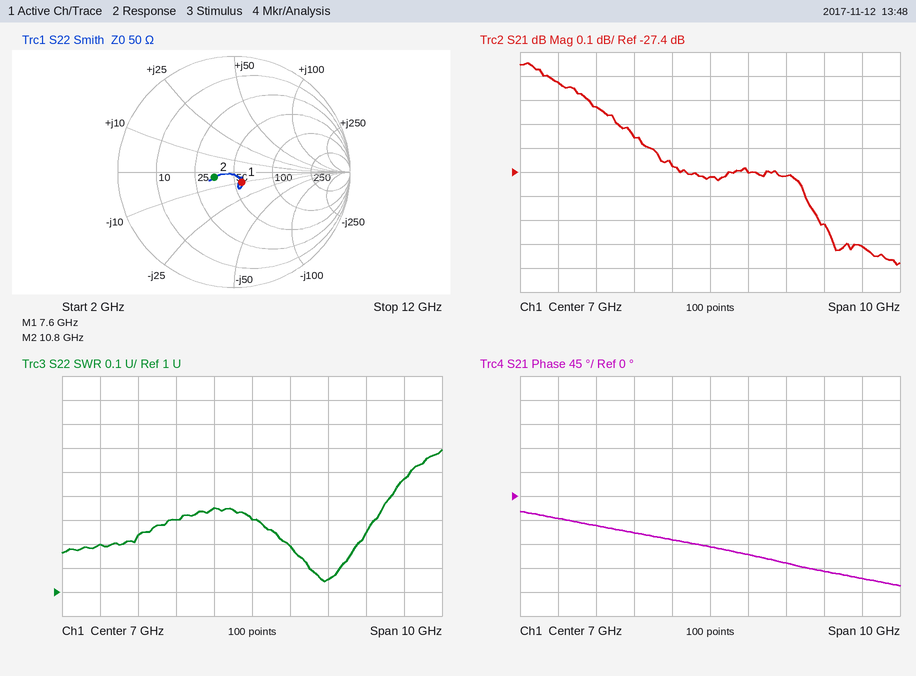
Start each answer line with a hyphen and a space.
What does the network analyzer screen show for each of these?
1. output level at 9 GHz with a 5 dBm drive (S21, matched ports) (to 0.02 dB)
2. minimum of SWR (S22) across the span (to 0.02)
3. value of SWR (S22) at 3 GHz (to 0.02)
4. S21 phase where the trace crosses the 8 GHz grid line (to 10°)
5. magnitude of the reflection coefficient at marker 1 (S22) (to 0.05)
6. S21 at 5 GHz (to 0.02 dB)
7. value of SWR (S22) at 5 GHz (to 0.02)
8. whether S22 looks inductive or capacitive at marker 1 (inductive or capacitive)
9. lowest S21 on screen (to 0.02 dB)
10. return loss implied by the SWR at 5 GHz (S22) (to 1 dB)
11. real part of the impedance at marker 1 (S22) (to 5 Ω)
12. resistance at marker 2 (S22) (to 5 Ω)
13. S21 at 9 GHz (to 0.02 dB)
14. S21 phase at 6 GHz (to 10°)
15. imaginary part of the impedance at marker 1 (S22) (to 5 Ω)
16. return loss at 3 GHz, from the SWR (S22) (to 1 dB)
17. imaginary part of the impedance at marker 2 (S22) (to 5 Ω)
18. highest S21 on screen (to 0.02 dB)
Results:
- -22.42 dBm
- 1.04
- 1.20
- -110°
- 0.10
- -27.26 dB
- 1.30
- capacitive
- -27.78 dB
- 18 dB
- 55 Ω
- 35 Ω
- -27.42 dB
- -80°
- -10 Ω
- 21 dB
- -5 Ω
- -26.94 dB
